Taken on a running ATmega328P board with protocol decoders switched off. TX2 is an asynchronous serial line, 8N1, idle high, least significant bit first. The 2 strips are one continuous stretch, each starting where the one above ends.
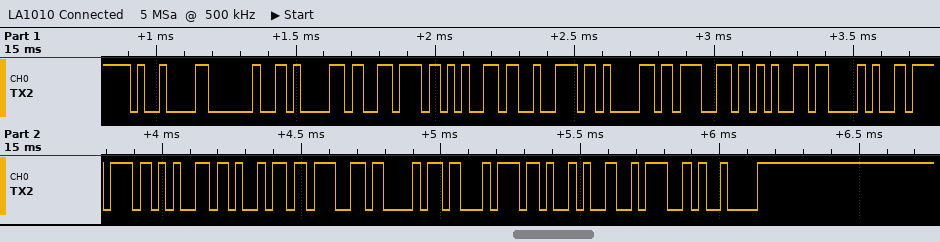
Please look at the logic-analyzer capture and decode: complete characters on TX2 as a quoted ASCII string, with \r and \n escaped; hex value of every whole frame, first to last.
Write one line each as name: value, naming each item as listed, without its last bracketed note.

complete characters on TX2 as a quoted ASCII string, with \r and \n escaped: "\t average(weight):\t"
hex value of every whole frame, first to last: 09 20 61 76 65 72 61 67 65 28 77 65 69 67 68 74 29 3A 09
